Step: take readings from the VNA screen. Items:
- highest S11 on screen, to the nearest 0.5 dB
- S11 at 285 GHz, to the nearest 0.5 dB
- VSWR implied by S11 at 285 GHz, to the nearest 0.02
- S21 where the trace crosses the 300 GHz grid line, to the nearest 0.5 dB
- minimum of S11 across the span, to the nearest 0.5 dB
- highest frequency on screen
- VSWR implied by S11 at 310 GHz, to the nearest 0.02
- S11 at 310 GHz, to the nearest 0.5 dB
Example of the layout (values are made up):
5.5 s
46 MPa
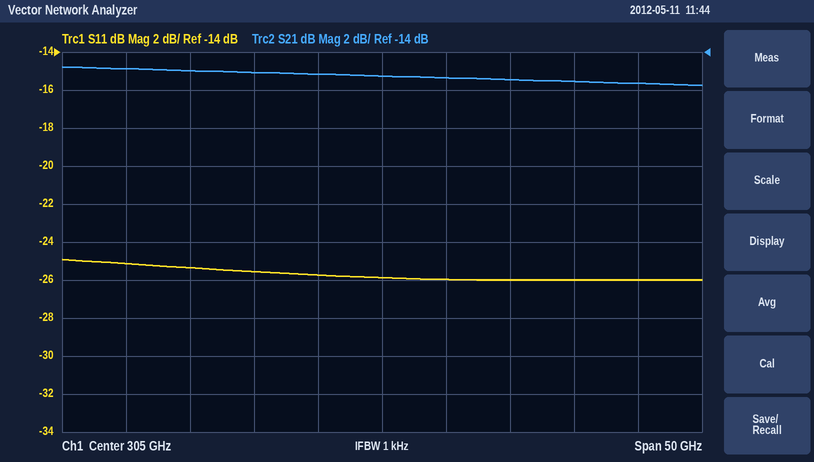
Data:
-25.0 dB
-25.0 dB
1.12
-15.0 dB
-26.0 dB
330 GHz
1.10
-26.0 dB
